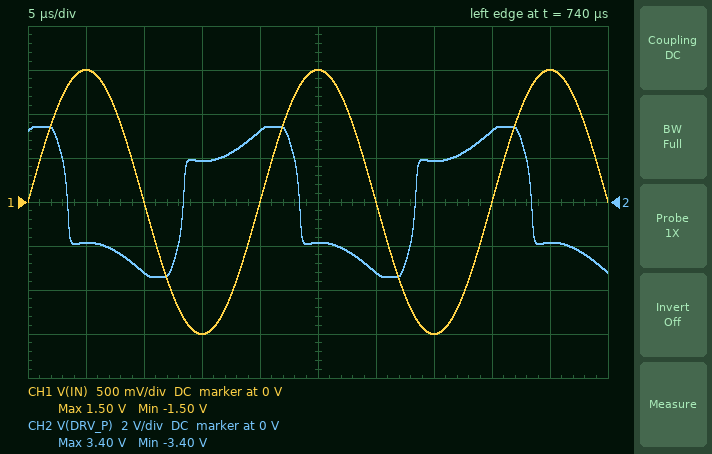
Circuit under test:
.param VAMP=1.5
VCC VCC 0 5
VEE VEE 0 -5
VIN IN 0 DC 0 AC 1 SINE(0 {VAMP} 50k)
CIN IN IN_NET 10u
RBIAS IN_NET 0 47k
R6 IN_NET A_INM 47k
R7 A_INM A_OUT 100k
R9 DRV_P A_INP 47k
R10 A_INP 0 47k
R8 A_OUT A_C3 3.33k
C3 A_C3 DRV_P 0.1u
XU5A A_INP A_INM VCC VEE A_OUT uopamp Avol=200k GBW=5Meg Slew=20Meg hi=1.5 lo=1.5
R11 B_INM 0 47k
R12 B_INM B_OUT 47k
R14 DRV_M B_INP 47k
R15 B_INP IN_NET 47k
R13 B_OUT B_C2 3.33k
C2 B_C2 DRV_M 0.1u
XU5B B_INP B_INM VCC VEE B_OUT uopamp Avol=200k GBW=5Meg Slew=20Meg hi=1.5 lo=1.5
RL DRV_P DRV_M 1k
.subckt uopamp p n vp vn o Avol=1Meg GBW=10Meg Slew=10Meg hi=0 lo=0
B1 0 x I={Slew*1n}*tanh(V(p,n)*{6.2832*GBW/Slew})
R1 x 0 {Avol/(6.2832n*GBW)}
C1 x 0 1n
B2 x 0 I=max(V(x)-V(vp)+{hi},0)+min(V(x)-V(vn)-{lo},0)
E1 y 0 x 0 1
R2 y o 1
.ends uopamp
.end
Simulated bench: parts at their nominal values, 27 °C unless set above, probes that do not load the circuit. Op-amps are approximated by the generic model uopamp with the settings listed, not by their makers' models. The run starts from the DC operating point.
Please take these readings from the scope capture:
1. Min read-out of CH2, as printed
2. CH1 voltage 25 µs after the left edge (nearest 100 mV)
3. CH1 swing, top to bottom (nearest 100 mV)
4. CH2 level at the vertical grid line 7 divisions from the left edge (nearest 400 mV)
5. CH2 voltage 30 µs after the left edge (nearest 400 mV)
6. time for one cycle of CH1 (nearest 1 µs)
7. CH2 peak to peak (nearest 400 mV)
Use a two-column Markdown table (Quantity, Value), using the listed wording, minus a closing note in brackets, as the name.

| Quantity | Value |
|---|---|
| Min read-out of CH2, as printed | -3.40 V |
| CH1 voltage 25 µs after the left edge | 1.5 V |
| CH1 swing, top to bottom | 3.0 V |
| CH2 level at the vertical grid line 7 divisions from the left edge | 2.0 V |
| CH2 voltage 30 µs after the left edge | -3.2 V |
| time for one cycle of CH1 | 20 µs |
| CH2 peak to peak | 6.8 V |
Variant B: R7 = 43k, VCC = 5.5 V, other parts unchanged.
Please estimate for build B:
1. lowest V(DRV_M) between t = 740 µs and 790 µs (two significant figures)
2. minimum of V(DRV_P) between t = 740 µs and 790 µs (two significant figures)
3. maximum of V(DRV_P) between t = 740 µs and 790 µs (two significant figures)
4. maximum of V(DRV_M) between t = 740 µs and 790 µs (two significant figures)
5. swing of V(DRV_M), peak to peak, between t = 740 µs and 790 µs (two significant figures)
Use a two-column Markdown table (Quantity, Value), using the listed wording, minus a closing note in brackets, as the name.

| Quantity | Value |
|---|---|
| lowest V(DRV_M) between t = 740 µs and 790 µs | -1.8 V |
| minimum of V(DRV_P) between t = 740 µs and 790 µs | -1.4 V |
| maximum of V(DRV_P) between t = 740 µs and 790 µs | 1.4 V |
| maximum of V(DRV_M) between t = 740 µs and 790 µs | 1.8 V |
| swing of V(DRV_M), peak to peak, between t = 740 µs and 790 µs | 3.6 V |
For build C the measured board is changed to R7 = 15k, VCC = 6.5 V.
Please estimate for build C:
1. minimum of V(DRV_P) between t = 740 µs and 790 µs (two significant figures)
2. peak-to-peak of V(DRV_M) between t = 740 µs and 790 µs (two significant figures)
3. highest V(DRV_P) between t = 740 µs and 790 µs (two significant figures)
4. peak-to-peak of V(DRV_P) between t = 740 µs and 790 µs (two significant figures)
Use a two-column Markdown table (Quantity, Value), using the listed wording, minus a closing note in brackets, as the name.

| Quantity | Value |
|---|---|
| minimum of V(DRV_P) between t = 740 µs and 790 µs | -2.0 V |
| peak-to-peak of V(DRV_M) between t = 740 µs and 790 µs | 5.3 V |
| highest V(DRV_P) between t = 740 µs and 790 µs | 2.5 V |
| peak-to-peak of V(DRV_P) between t = 740 µs and 790 µs | 4.5 V |
